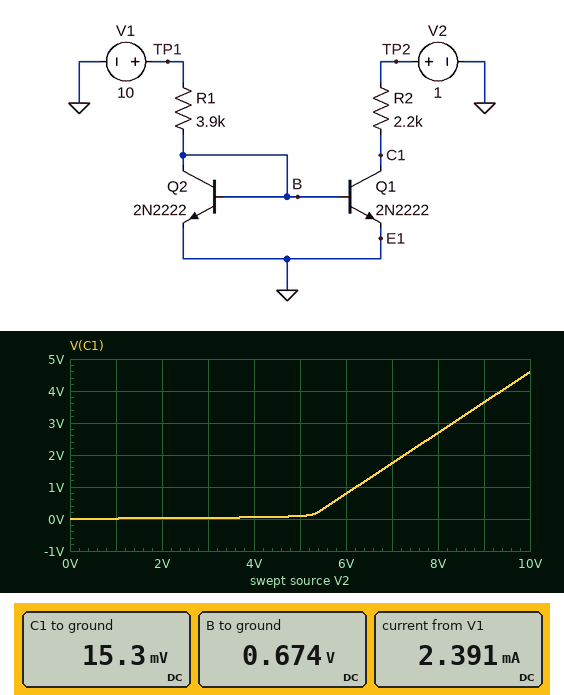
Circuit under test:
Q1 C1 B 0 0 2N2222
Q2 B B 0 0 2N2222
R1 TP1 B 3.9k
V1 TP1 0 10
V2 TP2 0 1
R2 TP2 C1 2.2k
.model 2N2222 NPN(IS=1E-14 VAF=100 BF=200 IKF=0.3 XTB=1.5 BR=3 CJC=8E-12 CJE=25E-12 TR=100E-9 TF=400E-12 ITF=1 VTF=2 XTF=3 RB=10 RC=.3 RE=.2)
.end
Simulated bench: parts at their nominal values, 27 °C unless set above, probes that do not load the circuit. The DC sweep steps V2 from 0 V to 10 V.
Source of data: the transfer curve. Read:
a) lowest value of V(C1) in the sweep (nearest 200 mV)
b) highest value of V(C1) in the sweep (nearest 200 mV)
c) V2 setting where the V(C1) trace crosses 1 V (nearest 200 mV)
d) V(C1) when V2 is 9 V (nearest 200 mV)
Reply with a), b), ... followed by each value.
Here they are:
a) 0 V
b) 4.6 V
c) 6.2 V
d) 3.6 V
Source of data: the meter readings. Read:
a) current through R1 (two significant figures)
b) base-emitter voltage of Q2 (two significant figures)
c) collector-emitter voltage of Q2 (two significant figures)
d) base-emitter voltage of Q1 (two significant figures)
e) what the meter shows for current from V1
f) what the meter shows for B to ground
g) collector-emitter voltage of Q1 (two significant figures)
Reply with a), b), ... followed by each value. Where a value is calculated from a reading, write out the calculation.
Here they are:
a) (10 V - 674 mV) / 3.9 kΩ = 2.4 mA
b) 674 mV = 670 mV
c) 674 mV = 670 mV
d) 674 mV = 670 mV
e) 2.391 mA
f) 0.674 V
g) 15.3 mV = 15 mV
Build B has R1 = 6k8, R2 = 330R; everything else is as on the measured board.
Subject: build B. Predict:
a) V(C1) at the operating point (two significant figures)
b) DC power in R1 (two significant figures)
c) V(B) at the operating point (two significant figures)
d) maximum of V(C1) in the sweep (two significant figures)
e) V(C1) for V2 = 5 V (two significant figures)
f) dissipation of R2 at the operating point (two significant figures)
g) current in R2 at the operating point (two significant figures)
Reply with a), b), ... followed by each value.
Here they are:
a) 550 mV
b) 13 mW
c) 660 mV
d) 9.5 V
e) 4.5 V
f) 610 µW
g) 1.4 mA
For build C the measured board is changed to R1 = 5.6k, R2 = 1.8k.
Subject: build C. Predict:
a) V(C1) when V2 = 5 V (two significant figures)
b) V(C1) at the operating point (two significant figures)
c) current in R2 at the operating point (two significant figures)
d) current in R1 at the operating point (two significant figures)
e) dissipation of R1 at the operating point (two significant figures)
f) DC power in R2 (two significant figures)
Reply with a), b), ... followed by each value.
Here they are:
a) 2.0 V
b) 21 mV
c) 540 µA
d) 1.7 mA
e) 16 mW
f) 530 µW
